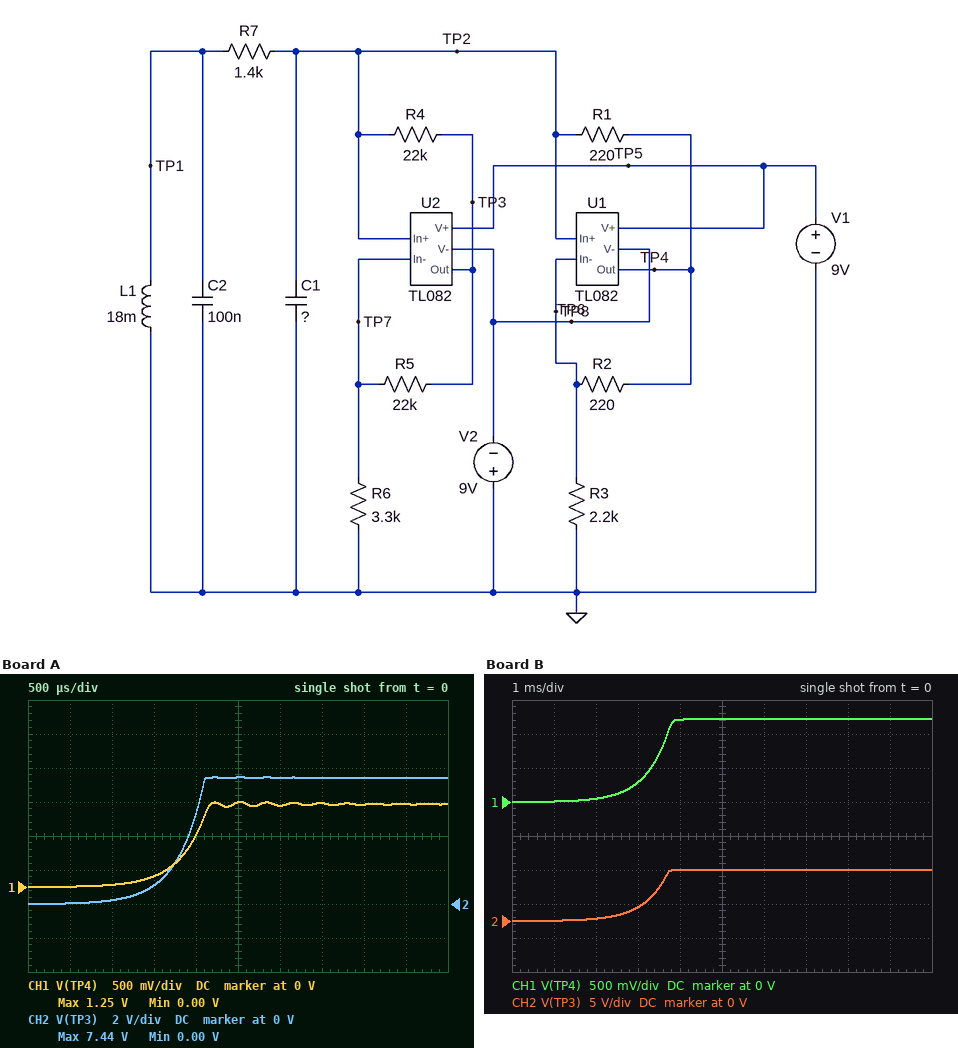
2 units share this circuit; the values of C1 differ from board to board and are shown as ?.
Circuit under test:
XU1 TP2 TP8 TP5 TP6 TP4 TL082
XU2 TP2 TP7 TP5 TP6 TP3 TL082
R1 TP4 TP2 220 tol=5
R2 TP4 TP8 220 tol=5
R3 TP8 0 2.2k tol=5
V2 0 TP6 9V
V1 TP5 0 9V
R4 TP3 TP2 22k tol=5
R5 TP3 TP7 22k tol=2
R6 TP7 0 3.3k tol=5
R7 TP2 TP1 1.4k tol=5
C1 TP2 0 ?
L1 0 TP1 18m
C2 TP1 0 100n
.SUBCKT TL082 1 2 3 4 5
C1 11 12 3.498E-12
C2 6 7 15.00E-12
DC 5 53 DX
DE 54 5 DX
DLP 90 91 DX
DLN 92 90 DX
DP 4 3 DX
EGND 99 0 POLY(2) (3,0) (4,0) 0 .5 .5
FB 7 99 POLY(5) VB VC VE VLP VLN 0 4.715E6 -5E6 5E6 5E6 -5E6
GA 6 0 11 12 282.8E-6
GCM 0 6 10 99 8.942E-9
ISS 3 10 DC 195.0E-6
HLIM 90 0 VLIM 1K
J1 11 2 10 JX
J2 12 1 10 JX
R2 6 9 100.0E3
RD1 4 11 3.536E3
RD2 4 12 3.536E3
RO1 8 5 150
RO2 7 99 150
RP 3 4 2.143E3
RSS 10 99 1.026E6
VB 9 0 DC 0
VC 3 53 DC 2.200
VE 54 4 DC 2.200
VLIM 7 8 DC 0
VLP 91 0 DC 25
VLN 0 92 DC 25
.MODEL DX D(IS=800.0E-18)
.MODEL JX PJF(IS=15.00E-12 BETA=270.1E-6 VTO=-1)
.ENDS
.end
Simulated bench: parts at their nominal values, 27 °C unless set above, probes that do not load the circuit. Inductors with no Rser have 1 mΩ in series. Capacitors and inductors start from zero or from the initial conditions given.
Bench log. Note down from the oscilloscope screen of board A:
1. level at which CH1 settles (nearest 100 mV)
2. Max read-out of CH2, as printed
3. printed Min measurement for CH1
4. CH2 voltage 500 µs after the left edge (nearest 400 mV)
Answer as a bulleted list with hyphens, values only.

- 1.2 V
- 7.44 V
- 0.00 V
- 0 V
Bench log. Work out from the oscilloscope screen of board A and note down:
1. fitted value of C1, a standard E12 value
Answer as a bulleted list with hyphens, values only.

- 22 nF
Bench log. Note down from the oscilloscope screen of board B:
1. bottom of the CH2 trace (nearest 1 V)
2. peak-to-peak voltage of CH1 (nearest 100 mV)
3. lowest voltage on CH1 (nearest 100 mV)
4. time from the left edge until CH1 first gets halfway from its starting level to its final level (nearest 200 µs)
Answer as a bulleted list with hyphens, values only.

- 0 V
- 1.2 V
- 0 V
- 3.4 ms
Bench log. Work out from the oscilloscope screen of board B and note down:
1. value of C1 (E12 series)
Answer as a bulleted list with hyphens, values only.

- 33 nF
